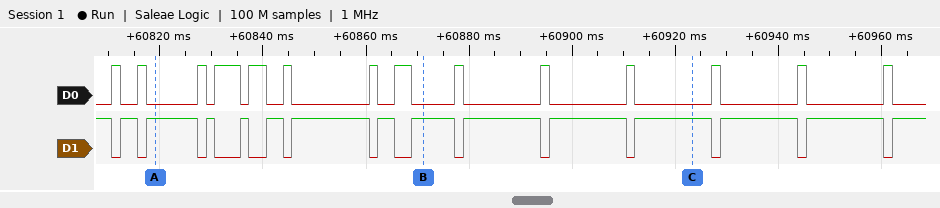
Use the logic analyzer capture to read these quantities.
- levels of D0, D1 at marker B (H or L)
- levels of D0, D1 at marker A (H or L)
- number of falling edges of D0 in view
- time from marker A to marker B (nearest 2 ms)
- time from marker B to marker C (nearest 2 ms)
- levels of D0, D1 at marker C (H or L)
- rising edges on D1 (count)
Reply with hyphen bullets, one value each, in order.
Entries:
- D0=L, D1=H
- D0=L, D1=H
- 14
- 52 ms
- 52 ms
- D0=L, D1=H
- 14
